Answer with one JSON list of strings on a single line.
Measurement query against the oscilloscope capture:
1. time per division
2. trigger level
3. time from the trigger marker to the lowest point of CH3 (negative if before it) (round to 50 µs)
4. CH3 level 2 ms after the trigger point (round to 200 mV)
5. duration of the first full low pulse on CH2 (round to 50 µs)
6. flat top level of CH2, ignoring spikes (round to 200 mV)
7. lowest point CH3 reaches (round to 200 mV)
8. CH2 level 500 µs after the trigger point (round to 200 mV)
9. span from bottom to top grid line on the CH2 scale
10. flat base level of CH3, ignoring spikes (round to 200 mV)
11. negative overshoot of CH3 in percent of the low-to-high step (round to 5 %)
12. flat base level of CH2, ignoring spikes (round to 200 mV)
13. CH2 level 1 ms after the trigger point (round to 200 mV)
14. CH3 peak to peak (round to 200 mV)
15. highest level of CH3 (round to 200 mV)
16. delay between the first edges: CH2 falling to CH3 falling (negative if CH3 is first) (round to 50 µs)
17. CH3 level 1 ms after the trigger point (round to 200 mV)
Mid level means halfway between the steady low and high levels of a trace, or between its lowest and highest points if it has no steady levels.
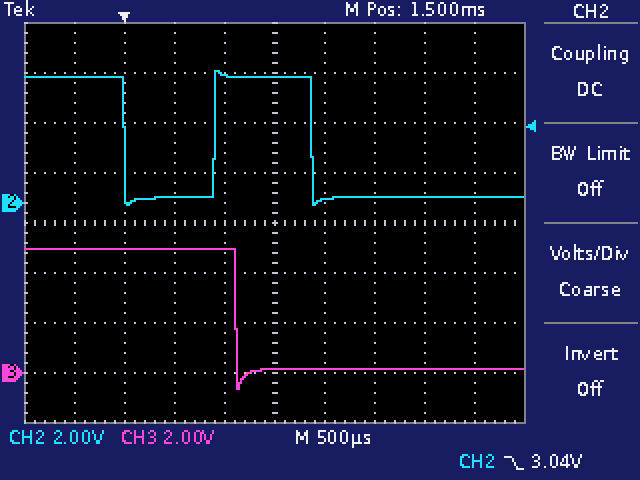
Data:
["500 µs", "3.04 V", "+1.15 ms", "200 mV", "900 µs", "5.0 V", "-600 mV", "200 mV", "16 V", "200 mV", "15 %", "200 mV", "5.2 V", "5.6 V", "5.0 V", "+1.10 ms", "5.0 V"]
